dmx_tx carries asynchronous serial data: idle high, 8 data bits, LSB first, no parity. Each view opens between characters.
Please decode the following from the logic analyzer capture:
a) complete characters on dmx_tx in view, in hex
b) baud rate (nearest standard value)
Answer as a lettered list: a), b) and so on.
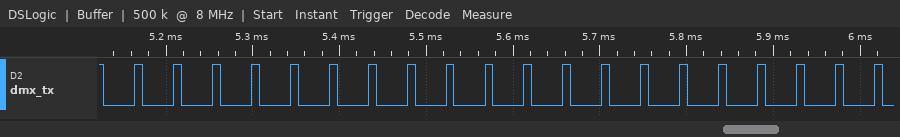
a) 08, 08, 08, 08, 08, 08, 08, 08, 08, 08
b) 115200 baud
